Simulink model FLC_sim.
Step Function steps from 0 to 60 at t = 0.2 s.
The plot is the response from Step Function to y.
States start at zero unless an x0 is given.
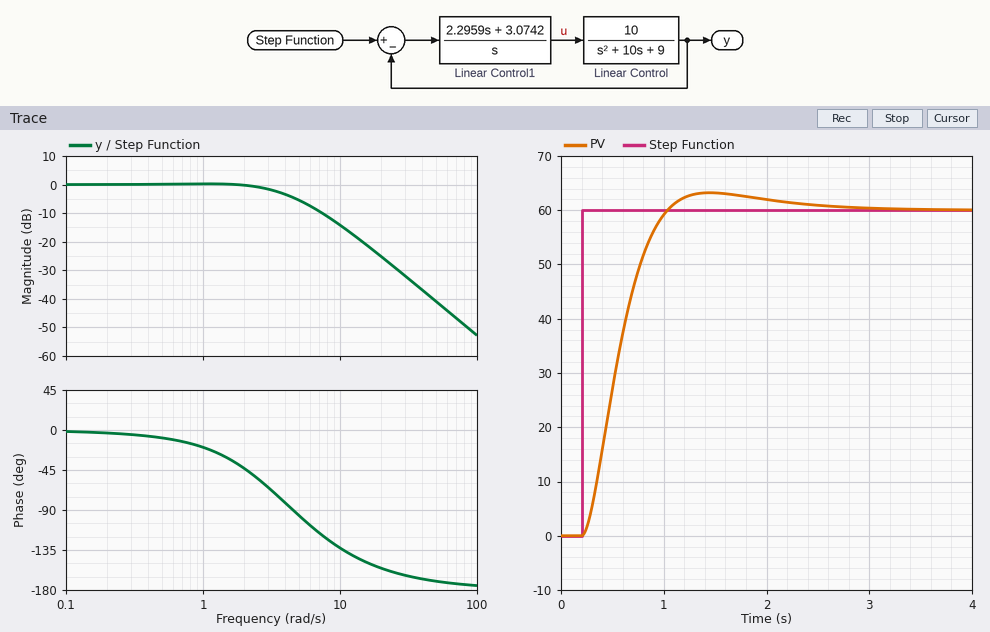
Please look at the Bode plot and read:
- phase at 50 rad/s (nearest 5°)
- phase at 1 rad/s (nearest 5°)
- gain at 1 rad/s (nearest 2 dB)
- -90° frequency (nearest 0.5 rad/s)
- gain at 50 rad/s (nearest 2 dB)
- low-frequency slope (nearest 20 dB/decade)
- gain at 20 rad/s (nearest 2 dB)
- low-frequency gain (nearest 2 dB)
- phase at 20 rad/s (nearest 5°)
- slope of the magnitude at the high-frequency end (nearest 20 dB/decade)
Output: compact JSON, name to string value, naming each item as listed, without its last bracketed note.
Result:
{"phase at 50 rad/s": "-170°", "phase at 1 rad/s": "-20°", "gain at 1 rad/s": "0 dB", "-90° frequency": "4.5 rad/s", "gain at 50 rad/s": "-40 dB", "low-frequency slope": "0 dB/decade", "gain at 20 rad/s": "-26 dB", "low-frequency gain": "0 dB", "phase at 20 rad/s": "-155°", "slope of the magnitude at the high-frequency end": "-40 dB/decade"}
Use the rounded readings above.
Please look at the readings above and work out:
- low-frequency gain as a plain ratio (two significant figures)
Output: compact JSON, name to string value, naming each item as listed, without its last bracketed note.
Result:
{"low-frequency gain as a plain ratio": "1.0"}
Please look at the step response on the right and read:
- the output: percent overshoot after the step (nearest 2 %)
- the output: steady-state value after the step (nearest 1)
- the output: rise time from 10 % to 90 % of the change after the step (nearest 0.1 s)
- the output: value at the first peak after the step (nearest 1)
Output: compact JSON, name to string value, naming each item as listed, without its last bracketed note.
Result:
{"the output: percent overshoot after the step": "6 %", "the output: steady-state value after the step": "60", "the output: rise time from 10 % to 90 % of the change after the step": "0.5 s", "the output: value at the first peak after the step": "63"}
